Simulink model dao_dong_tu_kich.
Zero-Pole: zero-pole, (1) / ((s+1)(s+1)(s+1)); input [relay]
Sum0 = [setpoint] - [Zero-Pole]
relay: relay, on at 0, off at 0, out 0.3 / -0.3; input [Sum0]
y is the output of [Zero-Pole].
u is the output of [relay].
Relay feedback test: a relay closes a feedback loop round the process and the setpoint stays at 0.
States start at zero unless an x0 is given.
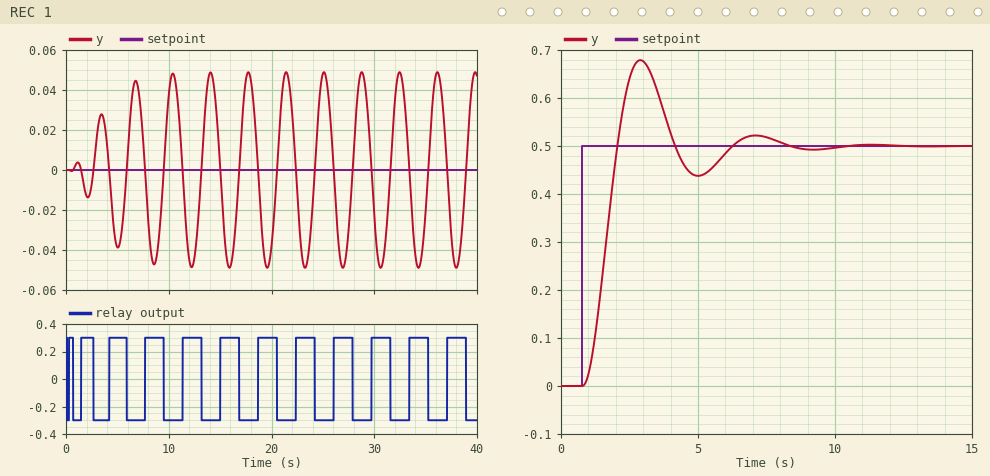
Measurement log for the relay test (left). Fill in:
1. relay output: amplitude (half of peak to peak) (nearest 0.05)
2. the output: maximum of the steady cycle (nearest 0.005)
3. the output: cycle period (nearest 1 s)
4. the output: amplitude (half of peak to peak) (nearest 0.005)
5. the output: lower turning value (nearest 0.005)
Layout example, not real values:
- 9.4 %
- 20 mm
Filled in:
- 0.30
- 0.050
- 4 s
- 0.050
- -0.050
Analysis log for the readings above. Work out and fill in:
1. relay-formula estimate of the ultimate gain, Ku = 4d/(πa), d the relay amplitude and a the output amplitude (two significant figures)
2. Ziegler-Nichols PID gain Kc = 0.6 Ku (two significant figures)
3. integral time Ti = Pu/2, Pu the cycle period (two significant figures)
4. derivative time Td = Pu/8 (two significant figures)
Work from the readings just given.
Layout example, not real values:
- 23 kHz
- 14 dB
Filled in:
- 7.6
- 4.6
- 2.0 s
- 0.50 s
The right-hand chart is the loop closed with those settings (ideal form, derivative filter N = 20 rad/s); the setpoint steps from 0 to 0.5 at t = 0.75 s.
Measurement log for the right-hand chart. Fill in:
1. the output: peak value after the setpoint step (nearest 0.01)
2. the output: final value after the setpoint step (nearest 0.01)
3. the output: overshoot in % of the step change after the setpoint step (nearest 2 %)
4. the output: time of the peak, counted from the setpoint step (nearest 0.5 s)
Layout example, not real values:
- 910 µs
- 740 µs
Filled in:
- 0.68
- 0.50
- 36 %
- 2.0 s
